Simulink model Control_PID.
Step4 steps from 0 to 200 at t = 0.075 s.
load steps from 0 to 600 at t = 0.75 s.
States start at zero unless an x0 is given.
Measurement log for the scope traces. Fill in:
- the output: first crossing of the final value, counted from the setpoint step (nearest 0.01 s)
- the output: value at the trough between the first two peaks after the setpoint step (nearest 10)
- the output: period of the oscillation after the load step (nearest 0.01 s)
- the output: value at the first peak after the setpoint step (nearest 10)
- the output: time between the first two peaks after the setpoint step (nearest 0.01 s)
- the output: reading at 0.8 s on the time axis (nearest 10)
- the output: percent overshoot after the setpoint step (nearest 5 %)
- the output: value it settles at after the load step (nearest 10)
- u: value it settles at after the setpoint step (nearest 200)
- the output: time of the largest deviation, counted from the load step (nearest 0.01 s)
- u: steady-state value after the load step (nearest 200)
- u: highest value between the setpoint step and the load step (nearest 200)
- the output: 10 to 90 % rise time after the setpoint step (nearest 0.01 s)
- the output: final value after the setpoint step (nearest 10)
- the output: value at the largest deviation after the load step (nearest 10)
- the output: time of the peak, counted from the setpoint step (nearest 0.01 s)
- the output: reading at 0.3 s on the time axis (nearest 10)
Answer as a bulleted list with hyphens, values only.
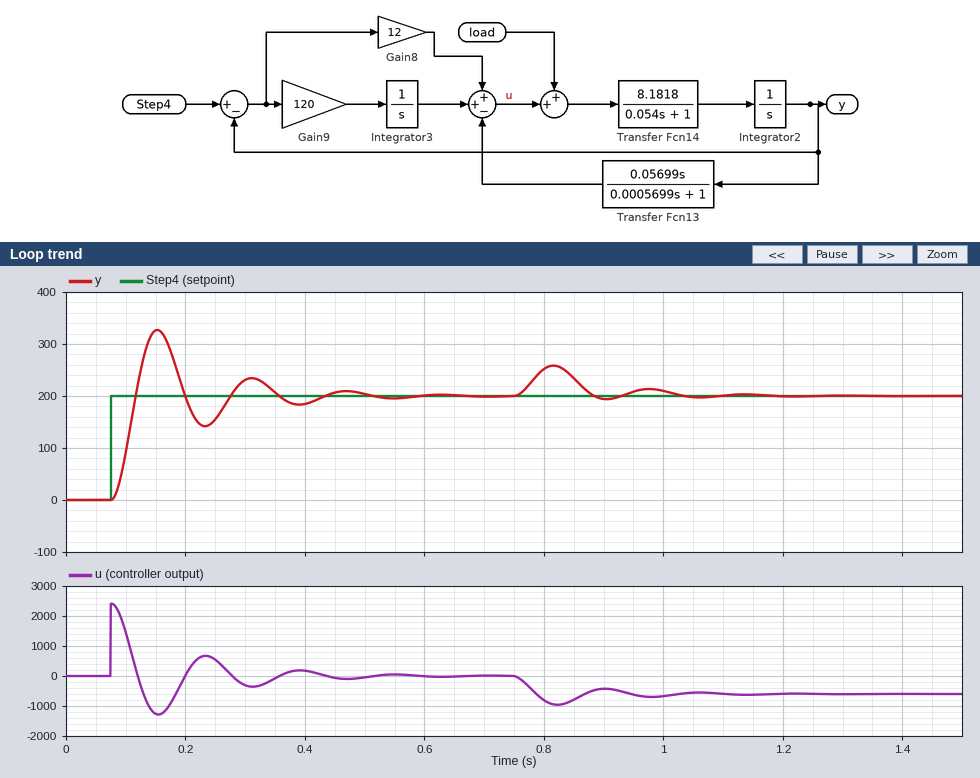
- 0.04 s
- 140
- 0.16 s
- 330
- 0.16 s
- 250
- 65 %
- 200
- 0
- 0.07 s
- -600
- 2400
- 0.03 s
- 200
- 260
- 0.08 s
- 230
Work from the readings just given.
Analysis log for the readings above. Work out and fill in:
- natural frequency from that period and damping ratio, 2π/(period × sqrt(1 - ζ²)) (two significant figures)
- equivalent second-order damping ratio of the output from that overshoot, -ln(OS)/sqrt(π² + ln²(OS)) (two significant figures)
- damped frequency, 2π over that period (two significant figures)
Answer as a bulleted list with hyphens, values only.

- 40 rad/s
- 0.14
- 39 rad/s
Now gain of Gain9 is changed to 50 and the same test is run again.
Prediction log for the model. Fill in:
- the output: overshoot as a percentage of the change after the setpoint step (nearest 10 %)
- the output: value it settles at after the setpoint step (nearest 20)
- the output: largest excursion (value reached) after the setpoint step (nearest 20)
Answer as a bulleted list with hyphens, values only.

- 50 %
- 200
- 300
